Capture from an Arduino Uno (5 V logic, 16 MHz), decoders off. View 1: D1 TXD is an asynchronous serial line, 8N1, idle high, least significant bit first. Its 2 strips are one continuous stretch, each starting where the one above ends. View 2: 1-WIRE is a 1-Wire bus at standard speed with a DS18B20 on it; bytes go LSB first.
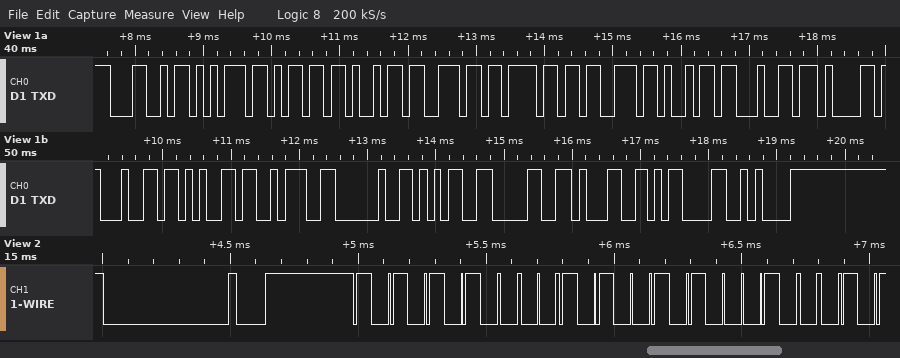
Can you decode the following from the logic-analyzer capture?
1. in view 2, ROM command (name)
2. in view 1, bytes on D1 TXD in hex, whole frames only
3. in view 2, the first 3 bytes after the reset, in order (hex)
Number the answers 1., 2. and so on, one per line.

1. Match ROM
2. 0x4C 0x75 0x6D 0x69 0x6E 0x6F 0x73 0x69 0x64 0x61 0x64 0x65 0x3A 0x20 0x35 0x30 0x31 0x0D 0x0A
3. 55 28 45
